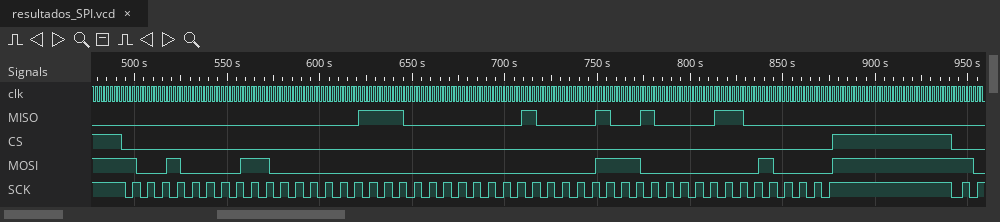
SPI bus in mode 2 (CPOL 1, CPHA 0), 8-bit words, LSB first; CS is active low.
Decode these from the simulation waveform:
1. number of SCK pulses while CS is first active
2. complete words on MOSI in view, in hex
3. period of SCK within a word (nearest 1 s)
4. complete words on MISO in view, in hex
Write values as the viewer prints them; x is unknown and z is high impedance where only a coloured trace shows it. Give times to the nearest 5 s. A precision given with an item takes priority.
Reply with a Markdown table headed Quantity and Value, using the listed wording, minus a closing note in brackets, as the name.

| Quantity | Value |
|---|---|
| number of SCK pulses while CS is first active | 48 |
| complete words on MOSI in view, in hex | 09, 03, 00, 00, 07, 08 |
| period of SCK within a word | 8 s |
| complete words on MISO in view, in hex | 00, 00, 07, 08, 09, 03 |
